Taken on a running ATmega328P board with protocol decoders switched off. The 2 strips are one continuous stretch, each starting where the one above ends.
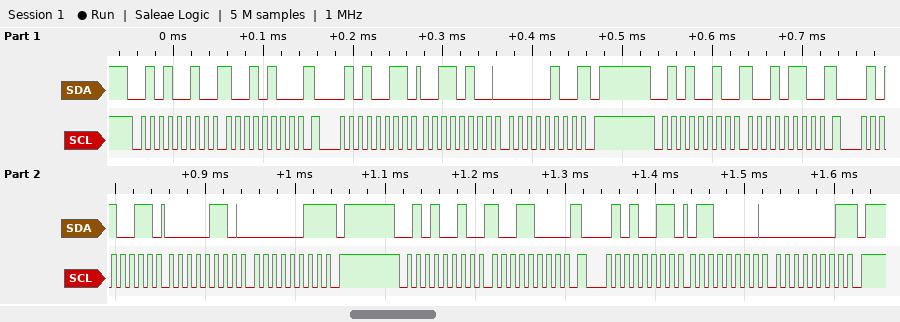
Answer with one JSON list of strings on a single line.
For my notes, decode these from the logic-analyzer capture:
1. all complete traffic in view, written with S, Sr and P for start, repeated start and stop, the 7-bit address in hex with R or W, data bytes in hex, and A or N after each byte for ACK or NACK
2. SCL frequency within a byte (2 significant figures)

["S 29W A 94 A Sr 29R A 34 A 04 N P S 29W A 96 A Sr 29R A 06 A 03 N P S 29W A 98 A Sr 29R A 60 A 01 N P", "100 kHz"]
